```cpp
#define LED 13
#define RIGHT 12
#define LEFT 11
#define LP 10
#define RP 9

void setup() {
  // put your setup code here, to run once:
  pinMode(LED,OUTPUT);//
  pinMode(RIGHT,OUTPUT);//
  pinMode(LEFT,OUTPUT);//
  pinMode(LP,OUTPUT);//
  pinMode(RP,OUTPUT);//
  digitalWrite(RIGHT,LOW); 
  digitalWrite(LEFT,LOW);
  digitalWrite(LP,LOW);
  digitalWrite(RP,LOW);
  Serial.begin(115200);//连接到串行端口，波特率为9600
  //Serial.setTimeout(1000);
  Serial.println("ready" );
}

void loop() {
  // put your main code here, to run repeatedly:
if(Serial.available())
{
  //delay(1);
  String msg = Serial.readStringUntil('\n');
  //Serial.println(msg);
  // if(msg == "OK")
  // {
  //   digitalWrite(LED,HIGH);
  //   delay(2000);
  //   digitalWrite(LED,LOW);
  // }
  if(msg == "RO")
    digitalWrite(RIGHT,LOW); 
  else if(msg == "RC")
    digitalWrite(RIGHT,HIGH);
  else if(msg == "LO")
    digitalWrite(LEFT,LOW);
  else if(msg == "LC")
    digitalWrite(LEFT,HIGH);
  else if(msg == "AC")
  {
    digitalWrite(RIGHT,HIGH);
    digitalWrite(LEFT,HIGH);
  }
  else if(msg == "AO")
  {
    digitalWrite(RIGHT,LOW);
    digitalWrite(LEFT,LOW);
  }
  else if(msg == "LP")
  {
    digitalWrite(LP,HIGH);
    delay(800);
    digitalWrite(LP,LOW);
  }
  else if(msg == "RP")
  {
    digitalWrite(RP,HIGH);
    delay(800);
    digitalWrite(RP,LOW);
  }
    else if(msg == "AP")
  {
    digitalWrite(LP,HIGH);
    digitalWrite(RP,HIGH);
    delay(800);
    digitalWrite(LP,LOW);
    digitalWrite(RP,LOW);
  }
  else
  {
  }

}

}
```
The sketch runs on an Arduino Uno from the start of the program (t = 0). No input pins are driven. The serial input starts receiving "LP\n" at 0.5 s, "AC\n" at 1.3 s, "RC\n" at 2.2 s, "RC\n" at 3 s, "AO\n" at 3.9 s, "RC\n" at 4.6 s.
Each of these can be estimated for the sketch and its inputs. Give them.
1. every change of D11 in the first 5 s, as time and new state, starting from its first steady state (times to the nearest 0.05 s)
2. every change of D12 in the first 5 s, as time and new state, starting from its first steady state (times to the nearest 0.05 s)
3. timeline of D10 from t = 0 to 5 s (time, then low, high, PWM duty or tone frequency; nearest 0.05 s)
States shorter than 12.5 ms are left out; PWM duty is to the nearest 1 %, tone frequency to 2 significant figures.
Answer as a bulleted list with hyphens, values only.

- 0 s low; 1.3 s high; 3.9 s low
- 0 s low; 1.3 s high; 3.9 s low; 4.6 s high
- 0 s low; 0.5 s high; 1.3 s low
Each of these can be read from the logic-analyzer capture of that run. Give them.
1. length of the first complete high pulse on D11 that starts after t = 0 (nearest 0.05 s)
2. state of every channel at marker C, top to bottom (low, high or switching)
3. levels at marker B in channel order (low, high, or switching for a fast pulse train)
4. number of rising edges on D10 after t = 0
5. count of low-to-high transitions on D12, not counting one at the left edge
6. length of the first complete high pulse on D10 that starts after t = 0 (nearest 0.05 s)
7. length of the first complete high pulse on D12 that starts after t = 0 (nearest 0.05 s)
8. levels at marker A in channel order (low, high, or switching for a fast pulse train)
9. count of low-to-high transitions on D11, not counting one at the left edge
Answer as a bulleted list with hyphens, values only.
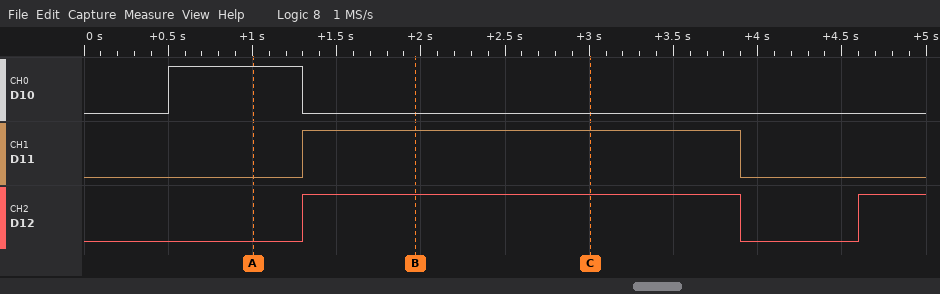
- 2.60 s
- D10 low, D11 high, D12 high
- D10 low, D11 high, D12 high
- 1
- 2
- 0.80 s
- 2.60 s
- D10 high, D11 low, D12 low
- 1
